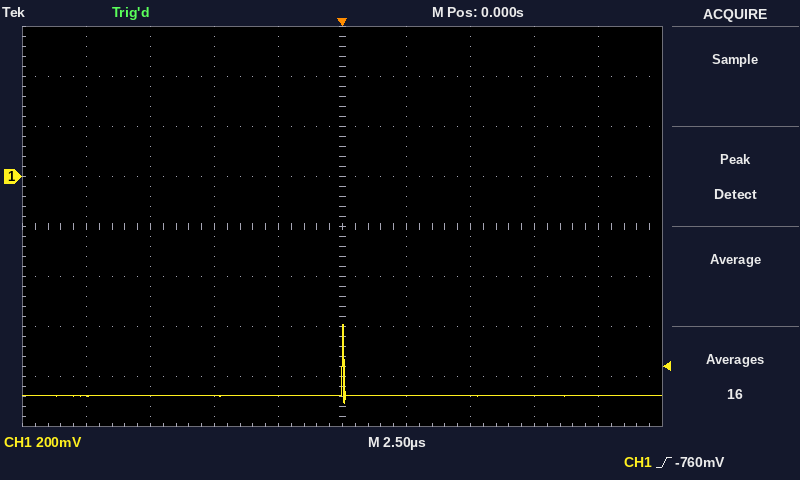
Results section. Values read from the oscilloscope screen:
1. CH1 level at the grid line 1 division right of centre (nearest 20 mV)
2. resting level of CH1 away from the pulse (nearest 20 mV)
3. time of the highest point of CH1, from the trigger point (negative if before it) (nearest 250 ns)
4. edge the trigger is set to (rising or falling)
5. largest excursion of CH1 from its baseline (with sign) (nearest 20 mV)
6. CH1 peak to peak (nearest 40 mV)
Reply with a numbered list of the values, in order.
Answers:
1. -880 mV
2. -880 mV
3. 0.00 µs
4. rising
5. +280 mV
6. 320 mV
